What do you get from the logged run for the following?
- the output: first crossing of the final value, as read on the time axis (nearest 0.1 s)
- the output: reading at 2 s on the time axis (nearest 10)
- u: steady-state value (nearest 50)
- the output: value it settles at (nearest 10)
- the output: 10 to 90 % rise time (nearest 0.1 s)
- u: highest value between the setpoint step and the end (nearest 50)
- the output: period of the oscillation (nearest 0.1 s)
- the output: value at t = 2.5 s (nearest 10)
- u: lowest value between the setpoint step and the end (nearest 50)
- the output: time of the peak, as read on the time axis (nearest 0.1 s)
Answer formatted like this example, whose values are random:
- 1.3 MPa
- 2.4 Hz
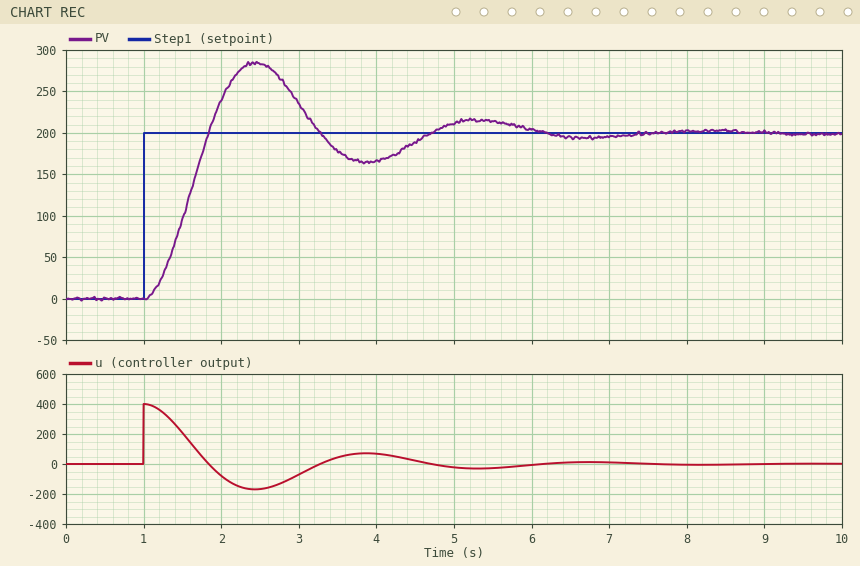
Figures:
- 1.8 s
- 240
- 0
- 200
- 0.6 s
- 400
- 2.9 s
- 280
- -150
- 2.4 s
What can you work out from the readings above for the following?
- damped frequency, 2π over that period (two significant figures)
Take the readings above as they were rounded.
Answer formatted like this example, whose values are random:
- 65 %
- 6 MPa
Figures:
- 2.2 rad/s
